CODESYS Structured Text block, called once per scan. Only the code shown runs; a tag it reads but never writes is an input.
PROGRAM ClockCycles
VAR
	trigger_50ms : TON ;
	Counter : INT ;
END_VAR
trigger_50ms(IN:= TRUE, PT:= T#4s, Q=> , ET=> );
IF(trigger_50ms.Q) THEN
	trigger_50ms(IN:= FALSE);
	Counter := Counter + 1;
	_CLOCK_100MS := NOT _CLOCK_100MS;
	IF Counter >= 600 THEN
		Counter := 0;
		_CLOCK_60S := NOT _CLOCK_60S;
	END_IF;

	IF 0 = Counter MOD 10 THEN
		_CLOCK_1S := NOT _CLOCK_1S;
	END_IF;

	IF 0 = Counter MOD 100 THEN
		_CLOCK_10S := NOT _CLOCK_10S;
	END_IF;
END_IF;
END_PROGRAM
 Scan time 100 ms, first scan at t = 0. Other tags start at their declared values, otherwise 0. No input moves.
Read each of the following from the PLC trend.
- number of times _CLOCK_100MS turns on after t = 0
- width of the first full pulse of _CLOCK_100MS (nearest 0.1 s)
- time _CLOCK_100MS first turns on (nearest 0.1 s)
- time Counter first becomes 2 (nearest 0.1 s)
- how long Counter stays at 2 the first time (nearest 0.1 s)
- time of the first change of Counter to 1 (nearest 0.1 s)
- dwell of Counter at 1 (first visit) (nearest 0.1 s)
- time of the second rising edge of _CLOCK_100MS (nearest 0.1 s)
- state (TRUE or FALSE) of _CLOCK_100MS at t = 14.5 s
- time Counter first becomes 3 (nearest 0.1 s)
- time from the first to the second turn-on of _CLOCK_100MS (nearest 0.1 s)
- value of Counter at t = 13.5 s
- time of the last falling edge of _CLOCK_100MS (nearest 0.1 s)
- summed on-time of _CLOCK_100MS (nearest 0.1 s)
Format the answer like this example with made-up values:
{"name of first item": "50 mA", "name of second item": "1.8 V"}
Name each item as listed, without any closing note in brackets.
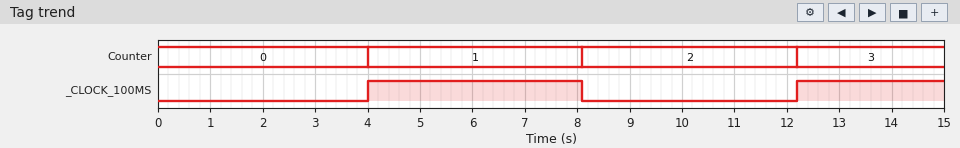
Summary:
{"number of times _CLOCK_100MS turns on after t = 0": "2", "width of the first full pulse of _CLOCK_100MS": "4.1 s", "time _CLOCK_100MS first turns on": "4.0 s", "time Counter first becomes 2": "8.1 s", "how long Counter stays at 2 the first time": "4.1 s", "time of the first change of Counter to 1": "4.0 s", "dwell of Counter at 1 (first visit)": "4.1 s", "time of the second rising edge of _CLOCK_100MS": "12.2 s", "state (TRUE or FALSE) of _CLOCK_100MS at t = 14.5 s": "TRUE", "time Counter first becomes 3": "12.2 s", "time from the first to the second turn-on of _CLOCK_100MS": "8.2 s", "value of Counter at t = 13.5 s": "3", "time of the last falling edge of _CLOCK_100MS": "8.1 s", "summed on-time of _CLOCK_100MS": "6.9 s"}
